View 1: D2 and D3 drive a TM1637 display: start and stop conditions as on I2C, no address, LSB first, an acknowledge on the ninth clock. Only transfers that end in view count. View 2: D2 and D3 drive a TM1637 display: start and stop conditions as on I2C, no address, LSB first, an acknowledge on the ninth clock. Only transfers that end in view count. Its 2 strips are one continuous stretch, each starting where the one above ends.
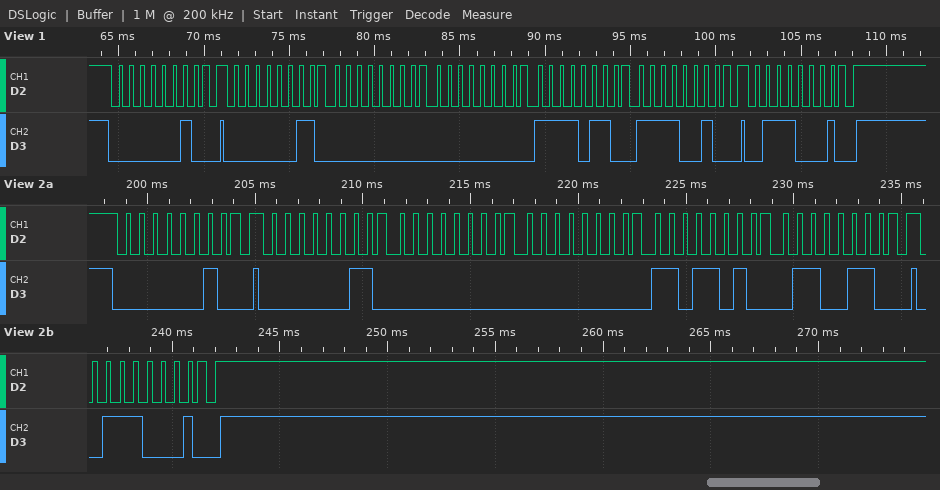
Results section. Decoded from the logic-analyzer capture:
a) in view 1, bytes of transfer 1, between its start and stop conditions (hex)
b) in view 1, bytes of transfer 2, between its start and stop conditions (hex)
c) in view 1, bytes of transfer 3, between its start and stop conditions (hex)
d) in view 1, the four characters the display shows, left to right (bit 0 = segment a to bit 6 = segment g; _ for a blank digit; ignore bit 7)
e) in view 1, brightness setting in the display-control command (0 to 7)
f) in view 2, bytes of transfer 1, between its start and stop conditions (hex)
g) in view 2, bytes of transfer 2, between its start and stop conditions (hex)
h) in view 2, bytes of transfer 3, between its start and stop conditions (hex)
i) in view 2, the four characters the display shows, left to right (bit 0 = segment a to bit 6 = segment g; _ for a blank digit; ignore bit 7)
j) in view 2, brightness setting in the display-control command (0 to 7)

40
C0 00 00 6F 4F
8E
__93
6
40
C0 00 00 5B 66
8E
__24
6
